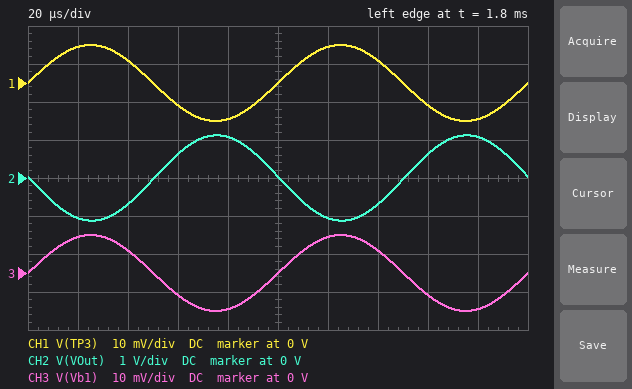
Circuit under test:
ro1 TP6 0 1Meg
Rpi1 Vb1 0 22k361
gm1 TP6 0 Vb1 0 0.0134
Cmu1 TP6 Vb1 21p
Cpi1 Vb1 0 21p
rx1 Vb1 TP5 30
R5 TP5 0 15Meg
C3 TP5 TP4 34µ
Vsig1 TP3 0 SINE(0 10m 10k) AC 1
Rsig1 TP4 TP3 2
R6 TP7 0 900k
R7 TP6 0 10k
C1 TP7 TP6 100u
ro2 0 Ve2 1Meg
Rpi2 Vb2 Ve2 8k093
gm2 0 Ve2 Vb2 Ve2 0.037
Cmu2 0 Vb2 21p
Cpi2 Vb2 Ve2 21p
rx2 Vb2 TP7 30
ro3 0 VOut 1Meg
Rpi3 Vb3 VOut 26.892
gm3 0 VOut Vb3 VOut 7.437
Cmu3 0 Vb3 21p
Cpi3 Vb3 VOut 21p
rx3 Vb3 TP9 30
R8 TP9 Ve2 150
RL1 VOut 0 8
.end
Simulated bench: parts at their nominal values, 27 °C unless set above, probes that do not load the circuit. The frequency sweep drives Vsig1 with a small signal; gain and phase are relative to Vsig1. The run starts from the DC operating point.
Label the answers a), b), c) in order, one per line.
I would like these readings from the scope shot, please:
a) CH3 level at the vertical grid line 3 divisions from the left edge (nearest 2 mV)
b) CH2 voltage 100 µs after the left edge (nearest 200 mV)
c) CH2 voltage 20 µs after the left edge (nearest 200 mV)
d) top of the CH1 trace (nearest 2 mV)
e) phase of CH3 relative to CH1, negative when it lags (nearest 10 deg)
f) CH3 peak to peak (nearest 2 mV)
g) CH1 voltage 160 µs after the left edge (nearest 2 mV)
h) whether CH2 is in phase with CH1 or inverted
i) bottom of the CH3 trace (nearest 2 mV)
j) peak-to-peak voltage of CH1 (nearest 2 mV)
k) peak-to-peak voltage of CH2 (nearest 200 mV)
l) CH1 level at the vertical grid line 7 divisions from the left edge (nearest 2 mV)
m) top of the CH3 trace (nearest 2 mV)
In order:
a) -6 mV
b) 0 V
c) -1.0 V
d) 10 mV
e) 0 deg
f) 20 mV
g) -6 mV
h) inverted
i) -10 mV
j) 20 mV
k) 2.2 V
l) 6 mV
m) 10 mV
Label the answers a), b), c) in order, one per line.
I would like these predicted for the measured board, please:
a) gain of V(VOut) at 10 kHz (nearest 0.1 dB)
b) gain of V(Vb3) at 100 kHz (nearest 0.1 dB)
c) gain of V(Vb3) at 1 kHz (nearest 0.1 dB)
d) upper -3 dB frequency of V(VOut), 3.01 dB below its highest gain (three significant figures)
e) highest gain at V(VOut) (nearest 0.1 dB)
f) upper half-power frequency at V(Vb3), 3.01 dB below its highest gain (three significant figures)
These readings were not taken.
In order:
a) 41.0 dB
b) 40.8 dB
c) 41.2 dB
d) 322 kHz
e) 41.0 dB
f) 322 kHz
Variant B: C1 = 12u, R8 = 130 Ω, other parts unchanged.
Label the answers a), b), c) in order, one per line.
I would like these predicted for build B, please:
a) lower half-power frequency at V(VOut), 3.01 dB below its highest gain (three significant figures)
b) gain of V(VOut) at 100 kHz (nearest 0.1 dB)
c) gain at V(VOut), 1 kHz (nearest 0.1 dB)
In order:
a) 216 mHz
b) 40.7 dB
c) 41.1 dB
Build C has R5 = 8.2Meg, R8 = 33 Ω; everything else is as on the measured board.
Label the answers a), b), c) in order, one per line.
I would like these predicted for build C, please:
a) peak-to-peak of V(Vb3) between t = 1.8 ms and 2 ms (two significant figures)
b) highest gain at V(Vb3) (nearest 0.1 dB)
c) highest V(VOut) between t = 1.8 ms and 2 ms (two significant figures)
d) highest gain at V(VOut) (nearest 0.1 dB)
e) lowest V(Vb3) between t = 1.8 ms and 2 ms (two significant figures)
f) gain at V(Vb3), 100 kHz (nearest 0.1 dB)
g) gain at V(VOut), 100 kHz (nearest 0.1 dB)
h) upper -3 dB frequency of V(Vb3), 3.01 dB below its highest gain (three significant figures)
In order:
a) 2.4 V
b) 41.7 dB
c) 1.2 V
d) 41.6 dB
e) -1.2 V
f) 41.3 dB
g) 41.2 dB
h) 322 kHz
